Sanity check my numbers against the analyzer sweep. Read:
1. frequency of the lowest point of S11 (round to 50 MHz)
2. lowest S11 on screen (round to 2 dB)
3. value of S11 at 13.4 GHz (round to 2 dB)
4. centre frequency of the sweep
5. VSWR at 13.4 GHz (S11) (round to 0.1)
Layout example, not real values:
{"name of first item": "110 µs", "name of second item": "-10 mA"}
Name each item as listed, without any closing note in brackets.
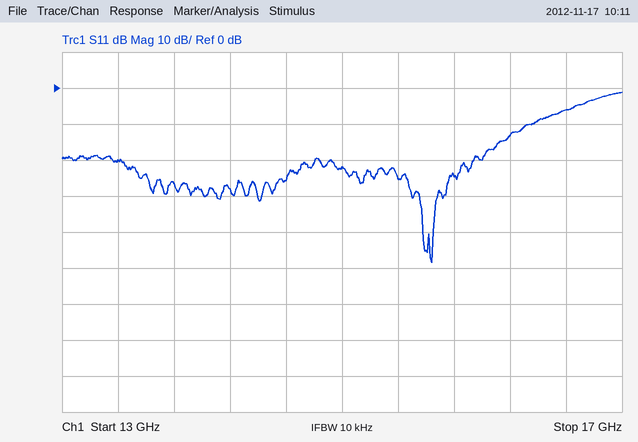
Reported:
{"frequency of the lowest point of S11": "15.65 GHz", "lowest S11 on screen": "-48 dB", "value of S11 at 13.4 GHz": "-20 dB", "centre frequency of the sweep": "15 GHz", "VSWR at 13.4 GHz (S11)": "1.2"}
